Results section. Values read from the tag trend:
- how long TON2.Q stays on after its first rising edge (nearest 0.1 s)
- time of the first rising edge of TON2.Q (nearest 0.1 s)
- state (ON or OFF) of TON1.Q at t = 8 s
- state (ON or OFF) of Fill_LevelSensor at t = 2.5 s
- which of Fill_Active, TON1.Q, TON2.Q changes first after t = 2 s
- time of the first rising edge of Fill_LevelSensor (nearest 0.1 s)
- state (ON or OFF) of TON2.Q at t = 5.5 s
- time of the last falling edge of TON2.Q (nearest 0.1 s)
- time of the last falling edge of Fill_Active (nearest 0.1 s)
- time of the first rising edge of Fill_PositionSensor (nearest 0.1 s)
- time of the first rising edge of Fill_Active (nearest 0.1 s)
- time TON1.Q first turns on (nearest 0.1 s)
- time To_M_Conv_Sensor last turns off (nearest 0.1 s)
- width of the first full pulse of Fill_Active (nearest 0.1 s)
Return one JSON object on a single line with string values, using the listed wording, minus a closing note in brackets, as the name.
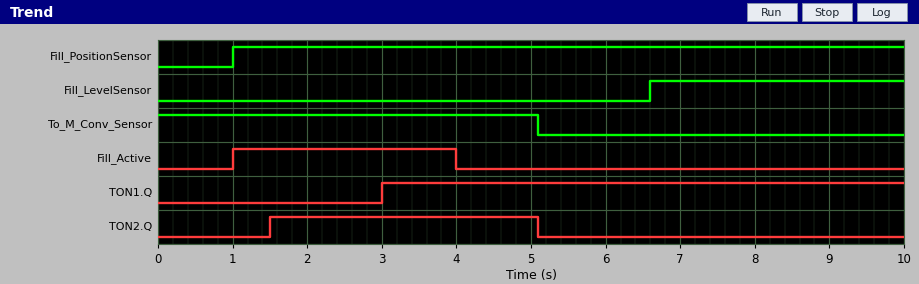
{"how long TON2.Q stays on after its first rising edge": "3.6 s", "time of the first rising edge of TON2.Q": "1.5 s", "state (ON or OFF) of TON1.Q at t = 8 s": "ON", "state (ON or OFF) of Fill_LevelSensor at t = 2.5 s": "OFF", "which of Fill_Active, TON1.Q, TON2.Q changes first after t = 2 s": "TON1.Q", "time of the first rising edge of Fill_LevelSensor": "6.6 s", "state (ON or OFF) of TON2.Q at t = 5.5 s": "OFF", "time of the last falling edge of TON2.Q": "5.1 s", "time of the last falling edge of Fill_Active": "4.0 s", "time of the first rising edge of Fill_PositionSensor": "1.0 s", "time of the first rising edge of Fill_Active": "1.0 s", "time TON1.Q first turns on": "3.0 s", "time To_M_Conv_Sensor last turns off": "5.1 s", "width of the first full pulse of Fill_Active": "3.0 s"}
